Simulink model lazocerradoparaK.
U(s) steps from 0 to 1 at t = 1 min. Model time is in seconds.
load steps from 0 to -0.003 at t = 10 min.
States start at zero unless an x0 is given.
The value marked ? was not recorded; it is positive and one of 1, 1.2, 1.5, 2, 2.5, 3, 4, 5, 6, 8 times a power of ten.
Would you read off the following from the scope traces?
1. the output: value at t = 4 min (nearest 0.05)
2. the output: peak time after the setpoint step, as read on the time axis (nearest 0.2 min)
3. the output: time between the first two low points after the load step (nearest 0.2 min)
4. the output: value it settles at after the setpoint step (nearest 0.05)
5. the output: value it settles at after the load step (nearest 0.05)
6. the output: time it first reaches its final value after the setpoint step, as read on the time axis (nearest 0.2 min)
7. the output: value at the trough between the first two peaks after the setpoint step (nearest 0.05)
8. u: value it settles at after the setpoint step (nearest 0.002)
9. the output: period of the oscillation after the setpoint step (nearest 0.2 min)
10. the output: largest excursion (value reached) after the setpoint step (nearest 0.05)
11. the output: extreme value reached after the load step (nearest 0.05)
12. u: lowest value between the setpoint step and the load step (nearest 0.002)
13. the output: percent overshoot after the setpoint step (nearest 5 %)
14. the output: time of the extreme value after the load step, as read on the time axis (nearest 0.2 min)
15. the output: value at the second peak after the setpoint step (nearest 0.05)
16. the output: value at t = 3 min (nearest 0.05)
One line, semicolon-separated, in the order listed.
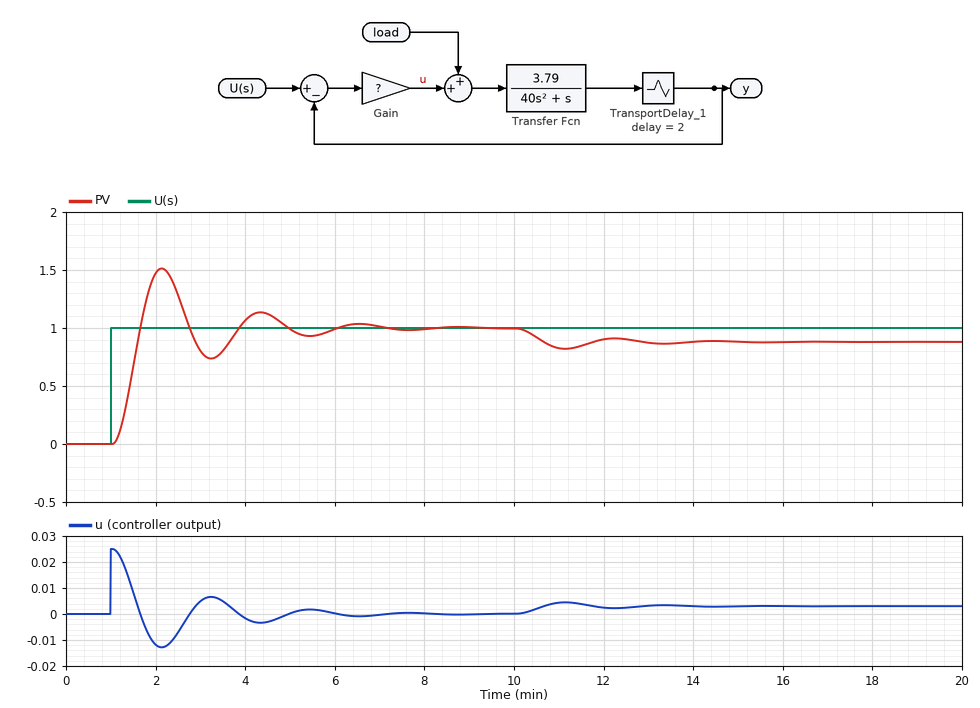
1.05; 2.2 min; 2.2 min; 1.00; 0.90; 1.6 min; 0.75; 0.000; 2.2 min; 1.50; 0.80; -0.012; 50 %; 11.2 min; 1.15; 0.80
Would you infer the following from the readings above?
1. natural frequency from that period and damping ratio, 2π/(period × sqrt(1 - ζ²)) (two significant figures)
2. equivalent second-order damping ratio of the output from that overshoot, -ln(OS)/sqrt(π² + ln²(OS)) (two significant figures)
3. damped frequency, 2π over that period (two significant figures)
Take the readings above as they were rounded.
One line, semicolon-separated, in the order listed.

2.9 rad/min; 0.22; 2.9 rad/min
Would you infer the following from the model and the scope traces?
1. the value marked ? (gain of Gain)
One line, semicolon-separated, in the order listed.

0.025
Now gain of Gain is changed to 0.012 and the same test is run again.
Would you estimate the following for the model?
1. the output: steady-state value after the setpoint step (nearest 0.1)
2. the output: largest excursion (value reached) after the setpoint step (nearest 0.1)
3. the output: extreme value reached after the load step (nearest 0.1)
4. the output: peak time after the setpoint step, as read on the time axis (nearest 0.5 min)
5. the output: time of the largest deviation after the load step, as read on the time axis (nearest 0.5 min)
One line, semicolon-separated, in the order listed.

1.0; 1.3; 0.7; 2.5 min; 11.5 min
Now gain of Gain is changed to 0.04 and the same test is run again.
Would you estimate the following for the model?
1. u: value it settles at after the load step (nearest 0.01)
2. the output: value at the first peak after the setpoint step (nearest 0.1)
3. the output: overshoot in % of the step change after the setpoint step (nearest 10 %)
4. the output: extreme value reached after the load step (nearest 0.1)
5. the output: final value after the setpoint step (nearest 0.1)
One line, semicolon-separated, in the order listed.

0.00; 1.6; 60 %; 0.9; 1.0
